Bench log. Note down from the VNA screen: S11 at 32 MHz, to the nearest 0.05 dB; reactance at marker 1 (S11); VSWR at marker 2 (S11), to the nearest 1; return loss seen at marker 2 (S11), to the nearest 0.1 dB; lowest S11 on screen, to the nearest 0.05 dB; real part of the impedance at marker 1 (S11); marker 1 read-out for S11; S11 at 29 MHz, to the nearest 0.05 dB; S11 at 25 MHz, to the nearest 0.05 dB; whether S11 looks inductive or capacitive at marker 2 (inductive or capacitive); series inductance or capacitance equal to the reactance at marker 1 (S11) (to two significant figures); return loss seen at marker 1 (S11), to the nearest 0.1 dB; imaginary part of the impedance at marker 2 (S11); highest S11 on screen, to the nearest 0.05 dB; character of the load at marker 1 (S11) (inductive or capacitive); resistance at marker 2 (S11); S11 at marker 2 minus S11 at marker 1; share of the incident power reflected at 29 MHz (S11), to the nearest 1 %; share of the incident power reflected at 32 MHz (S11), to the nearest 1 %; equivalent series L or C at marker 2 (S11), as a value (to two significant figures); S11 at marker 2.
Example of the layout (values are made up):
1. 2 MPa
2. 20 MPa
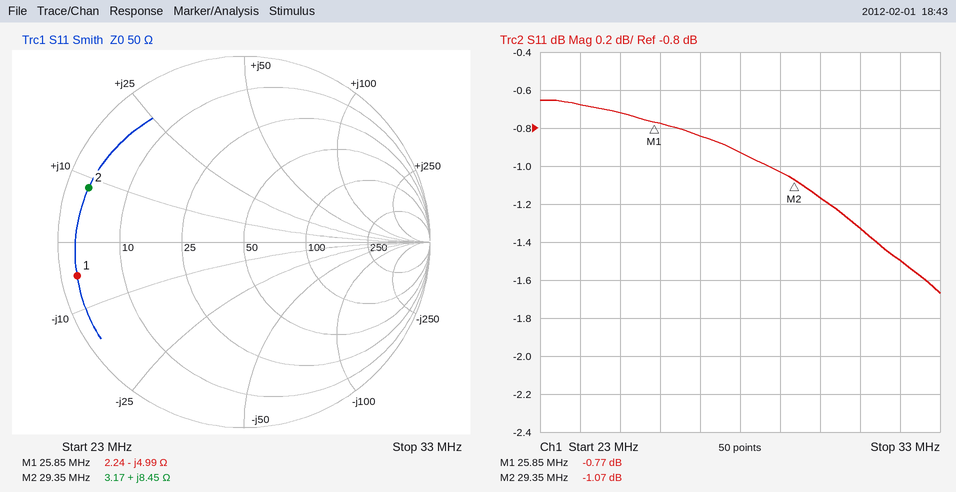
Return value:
1. -1.50 dB
2. -4.99 Ω
3. 16
4. 1.1 dB
5. -1.65 dB
6. 2.24 Ω
7. -0.77 dB
8. -1.05 dB
9. -0.70 dB
10. inductive
11. 1.2 nF
12. 0.8 dB
13. +8.45 Ω
14. -0.65 dB
15. capacitive
16. 3.17 Ω
17. -0.30 dB
18. 79 %
19. 71 %
20. 46 nH
21. -1.07 dB
